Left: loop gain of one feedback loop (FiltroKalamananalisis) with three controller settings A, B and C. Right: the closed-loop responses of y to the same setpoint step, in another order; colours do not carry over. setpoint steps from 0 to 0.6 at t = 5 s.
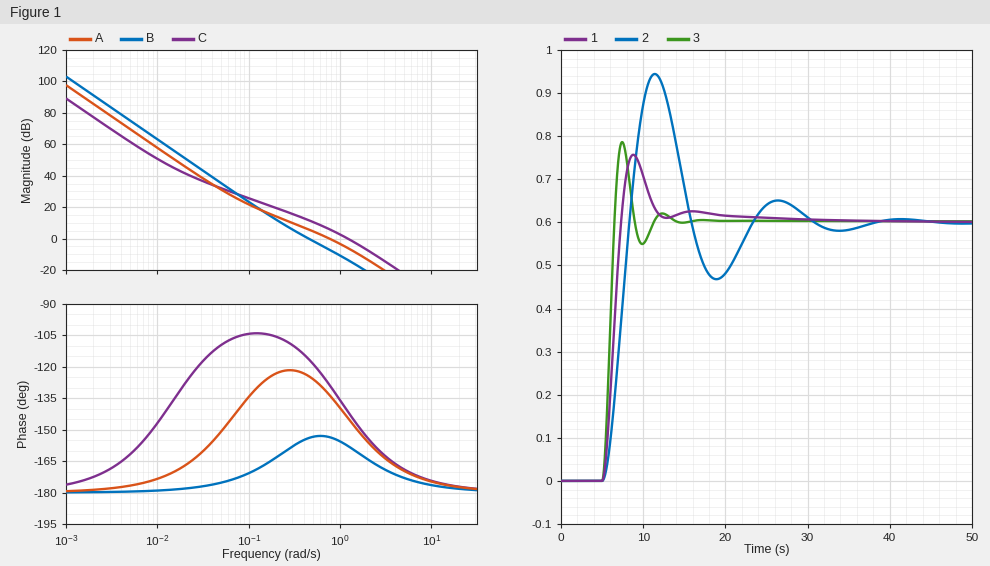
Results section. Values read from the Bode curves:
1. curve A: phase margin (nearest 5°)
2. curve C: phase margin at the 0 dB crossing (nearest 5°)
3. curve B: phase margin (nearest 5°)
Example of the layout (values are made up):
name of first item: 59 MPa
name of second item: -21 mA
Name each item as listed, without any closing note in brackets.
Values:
curve A: phase margin: 45°
curve C: phase margin at the 0 dB crossing: 40°
curve B: phase margin: 25°
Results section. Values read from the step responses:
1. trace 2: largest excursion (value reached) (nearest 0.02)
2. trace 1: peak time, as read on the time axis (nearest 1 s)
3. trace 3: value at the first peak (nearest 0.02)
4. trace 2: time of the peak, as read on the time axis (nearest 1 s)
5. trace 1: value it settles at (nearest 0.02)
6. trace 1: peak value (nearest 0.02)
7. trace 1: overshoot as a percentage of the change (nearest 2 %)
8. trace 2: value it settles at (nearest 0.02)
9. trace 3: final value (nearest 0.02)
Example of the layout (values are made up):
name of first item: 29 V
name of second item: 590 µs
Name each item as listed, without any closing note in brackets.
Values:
trace 2: largest excursion (value reached): 0.94
trace 1: peak time, as read on the time axis: 9 s
trace 3: value at the first peak: 0.78
trace 2: time of the peak, as read on the time axis: 11 s
trace 1: value it settles at: 0.60
trace 1: peak value: 0.76
trace 1: overshoot as a percentage of the change: 26 %
trace 2: value it settles at: 0.60
trace 3: final value: 0.60
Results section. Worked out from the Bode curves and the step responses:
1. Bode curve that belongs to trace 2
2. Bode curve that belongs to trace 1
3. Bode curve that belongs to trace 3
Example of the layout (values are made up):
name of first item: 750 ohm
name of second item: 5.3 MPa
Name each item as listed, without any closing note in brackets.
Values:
Bode curve that belongs to trace 2: B
Bode curve that belongs to trace 1: A
Bode curve that belongs to trace 3: C
